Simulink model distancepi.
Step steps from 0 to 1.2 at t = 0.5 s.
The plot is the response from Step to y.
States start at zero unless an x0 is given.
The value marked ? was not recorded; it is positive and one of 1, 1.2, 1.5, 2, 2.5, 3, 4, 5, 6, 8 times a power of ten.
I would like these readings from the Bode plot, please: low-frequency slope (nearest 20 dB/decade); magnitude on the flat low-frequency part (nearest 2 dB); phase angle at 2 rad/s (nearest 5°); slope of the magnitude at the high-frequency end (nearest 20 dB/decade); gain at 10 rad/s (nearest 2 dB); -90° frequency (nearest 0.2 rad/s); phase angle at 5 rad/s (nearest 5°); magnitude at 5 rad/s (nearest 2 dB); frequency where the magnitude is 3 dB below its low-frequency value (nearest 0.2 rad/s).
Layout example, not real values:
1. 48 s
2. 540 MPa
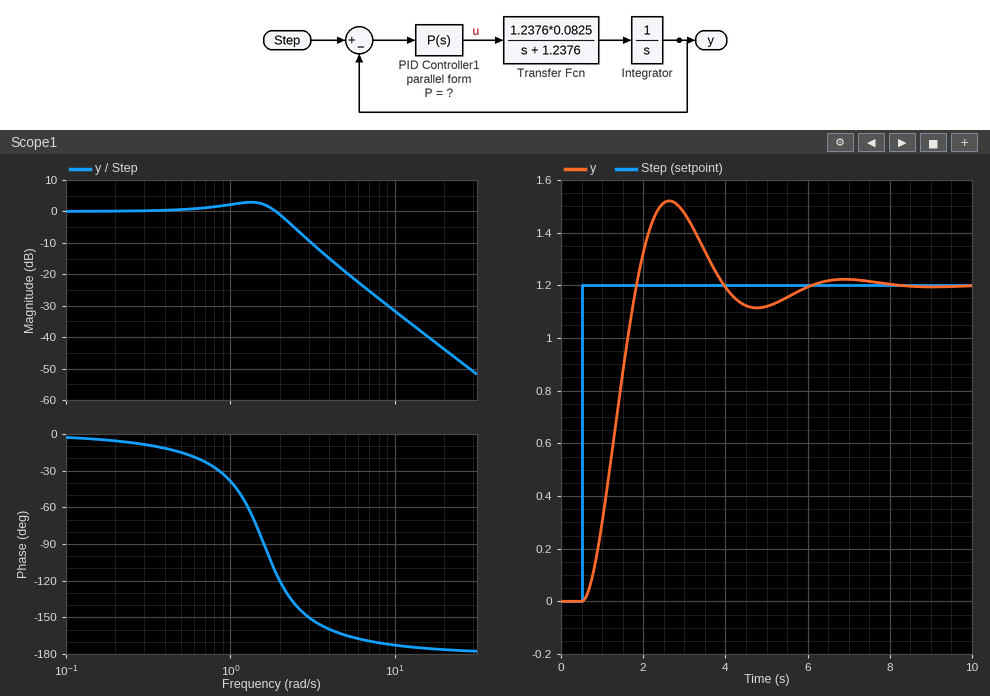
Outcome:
1. 0 dB/decade
2. 0 dB
3. -120°
4. -40 dB/decade
5. -32 dB
6. 1.6 rad/s
7. -165°
8. -20 dB
9. 2.2 rad/s
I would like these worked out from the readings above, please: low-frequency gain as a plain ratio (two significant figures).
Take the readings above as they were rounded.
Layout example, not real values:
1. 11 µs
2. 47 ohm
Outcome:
1. 1.0
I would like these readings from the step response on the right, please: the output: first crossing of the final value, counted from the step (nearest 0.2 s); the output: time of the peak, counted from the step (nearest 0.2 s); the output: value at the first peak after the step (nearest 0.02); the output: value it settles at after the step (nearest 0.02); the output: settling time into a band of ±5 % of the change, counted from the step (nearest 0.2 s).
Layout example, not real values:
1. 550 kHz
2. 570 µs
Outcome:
1. 1.4 s
2. 2.2 s
3. 1.52
4. 1.20
5. 4.8 s
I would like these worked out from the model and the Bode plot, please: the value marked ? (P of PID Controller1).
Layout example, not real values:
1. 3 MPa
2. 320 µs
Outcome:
1. 25
